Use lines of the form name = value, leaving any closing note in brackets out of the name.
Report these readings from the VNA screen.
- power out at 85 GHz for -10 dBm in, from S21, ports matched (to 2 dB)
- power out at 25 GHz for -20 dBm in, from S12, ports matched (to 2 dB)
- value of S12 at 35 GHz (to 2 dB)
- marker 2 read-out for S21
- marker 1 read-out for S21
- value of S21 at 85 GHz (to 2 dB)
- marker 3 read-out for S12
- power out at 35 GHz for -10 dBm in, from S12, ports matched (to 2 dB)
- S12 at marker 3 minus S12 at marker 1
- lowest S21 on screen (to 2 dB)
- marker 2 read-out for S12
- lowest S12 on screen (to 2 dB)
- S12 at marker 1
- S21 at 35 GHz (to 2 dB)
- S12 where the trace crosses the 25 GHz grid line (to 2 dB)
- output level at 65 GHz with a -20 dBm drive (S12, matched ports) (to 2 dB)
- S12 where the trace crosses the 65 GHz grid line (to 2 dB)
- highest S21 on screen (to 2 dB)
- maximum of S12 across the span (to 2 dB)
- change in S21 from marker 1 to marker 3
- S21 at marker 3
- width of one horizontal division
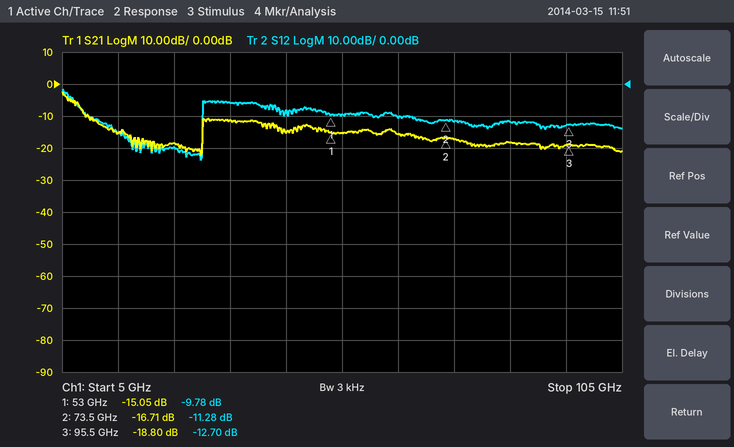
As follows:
power out at 85 GHz for -10 dBm in, from S21, ports matched = -28 dBm
power out at 25 GHz for -20 dBm in, from S12, ports matched = -40 dBm
value of S12 at 35 GHz = -6 dB
marker 2 read-out for S21 = -16.71 dB
marker 1 read-out for S21 = -15.05 dB
value of S21 at 85 GHz = -18 dB
marker 3 read-out for S12 = -12.70 dB
power out at 35 GHz for -10 dBm in, from S12, ports matched = -16 dBm
S12 at marker 3 minus S12 at marker 1 = -2.92 dB
lowest S21 on screen = -22 dB
marker 2 read-out for S12 = -11.28 dB
lowest S12 on screen = -24 dB
S12 at marker 1 = -9.78 dB
S21 at 35 GHz = -12 dB
S12 where the trace crosses the 25 GHz grid line = -20 dB
output level at 65 GHz with a -20 dBm drive (S12, matched ports) = -30 dBm
S12 where the trace crosses the 65 GHz grid line = -10 dB
highest S21 on screen = -2 dB
maximum of S12 across the span = -2 dB
change in S21 from marker 1 to marker 3 = -3.75 dB
S21 at marker 3 = -18.80 dB
width of one horizontal division = 10 GHz
